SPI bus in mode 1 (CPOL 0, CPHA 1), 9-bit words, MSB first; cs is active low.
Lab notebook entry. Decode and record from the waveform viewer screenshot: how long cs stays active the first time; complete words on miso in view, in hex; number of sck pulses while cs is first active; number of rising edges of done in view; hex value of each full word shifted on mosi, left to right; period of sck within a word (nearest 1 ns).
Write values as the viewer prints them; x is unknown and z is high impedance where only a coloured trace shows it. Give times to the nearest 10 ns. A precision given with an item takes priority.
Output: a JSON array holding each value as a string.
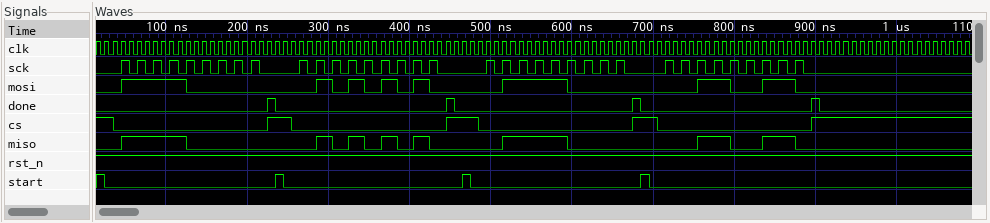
["190 ns", "1E0, 0AA, 0F0, 066", "9", "4", "1E0, 0AA, 0F0, 066", "20 ns"]
